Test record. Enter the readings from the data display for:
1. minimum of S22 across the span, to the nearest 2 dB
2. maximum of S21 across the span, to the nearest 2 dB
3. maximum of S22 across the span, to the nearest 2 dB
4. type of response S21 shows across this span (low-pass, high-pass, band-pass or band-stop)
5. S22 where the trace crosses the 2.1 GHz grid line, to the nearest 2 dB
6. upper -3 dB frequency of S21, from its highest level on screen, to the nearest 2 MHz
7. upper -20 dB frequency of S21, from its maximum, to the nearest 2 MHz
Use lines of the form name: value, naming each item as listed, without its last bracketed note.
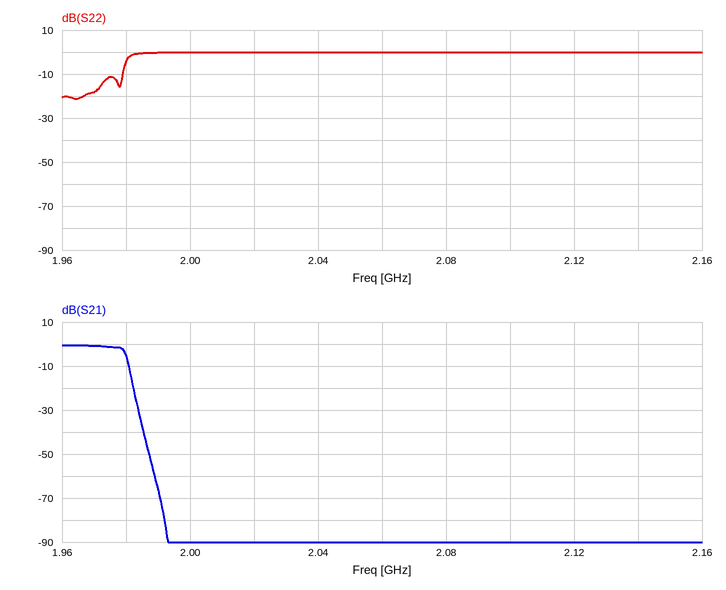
minimum of S22 across the span, to the nearest 2 dB: -22 dB
maximum of S21 across the span, to the nearest 2 dB: 0 dB
maximum of S22 across the span, to the nearest 2 dB: 0 dB
type of response S21 shows across this span: low-pass
S22 where the trace crosses the 2.1 GHz grid line, to the nearest 2 dB: 0 dB
upper -3 dB frequency of S21, from its highest level on screen, to the nearest 2 MHz: 1.980 GHz
upper -20 dB frequency of S21, from its maximum, to the nearest 2 MHz: 1.982 GHz
